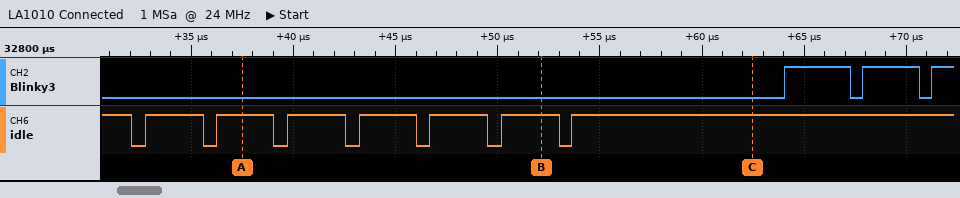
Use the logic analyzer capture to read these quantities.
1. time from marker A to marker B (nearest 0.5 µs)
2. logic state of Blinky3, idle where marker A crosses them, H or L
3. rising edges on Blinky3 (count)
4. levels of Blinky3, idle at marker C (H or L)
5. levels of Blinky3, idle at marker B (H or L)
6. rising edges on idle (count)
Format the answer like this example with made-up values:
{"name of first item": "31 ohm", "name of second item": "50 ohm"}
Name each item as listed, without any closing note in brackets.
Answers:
{"time from marker A to marker B": "14.5 µs", "logic state of Blinky3, idle where marker A crosses them, H or L": "Blinky3=L, idle=H", "rising edges on Blinky3": "3", "levels of Blinky3, idle at marker C": "Blinky3=L, idle=H", "levels of Blinky3, idle at marker B": "Blinky3=L, idle=H", "rising edges on idle": "7"}
